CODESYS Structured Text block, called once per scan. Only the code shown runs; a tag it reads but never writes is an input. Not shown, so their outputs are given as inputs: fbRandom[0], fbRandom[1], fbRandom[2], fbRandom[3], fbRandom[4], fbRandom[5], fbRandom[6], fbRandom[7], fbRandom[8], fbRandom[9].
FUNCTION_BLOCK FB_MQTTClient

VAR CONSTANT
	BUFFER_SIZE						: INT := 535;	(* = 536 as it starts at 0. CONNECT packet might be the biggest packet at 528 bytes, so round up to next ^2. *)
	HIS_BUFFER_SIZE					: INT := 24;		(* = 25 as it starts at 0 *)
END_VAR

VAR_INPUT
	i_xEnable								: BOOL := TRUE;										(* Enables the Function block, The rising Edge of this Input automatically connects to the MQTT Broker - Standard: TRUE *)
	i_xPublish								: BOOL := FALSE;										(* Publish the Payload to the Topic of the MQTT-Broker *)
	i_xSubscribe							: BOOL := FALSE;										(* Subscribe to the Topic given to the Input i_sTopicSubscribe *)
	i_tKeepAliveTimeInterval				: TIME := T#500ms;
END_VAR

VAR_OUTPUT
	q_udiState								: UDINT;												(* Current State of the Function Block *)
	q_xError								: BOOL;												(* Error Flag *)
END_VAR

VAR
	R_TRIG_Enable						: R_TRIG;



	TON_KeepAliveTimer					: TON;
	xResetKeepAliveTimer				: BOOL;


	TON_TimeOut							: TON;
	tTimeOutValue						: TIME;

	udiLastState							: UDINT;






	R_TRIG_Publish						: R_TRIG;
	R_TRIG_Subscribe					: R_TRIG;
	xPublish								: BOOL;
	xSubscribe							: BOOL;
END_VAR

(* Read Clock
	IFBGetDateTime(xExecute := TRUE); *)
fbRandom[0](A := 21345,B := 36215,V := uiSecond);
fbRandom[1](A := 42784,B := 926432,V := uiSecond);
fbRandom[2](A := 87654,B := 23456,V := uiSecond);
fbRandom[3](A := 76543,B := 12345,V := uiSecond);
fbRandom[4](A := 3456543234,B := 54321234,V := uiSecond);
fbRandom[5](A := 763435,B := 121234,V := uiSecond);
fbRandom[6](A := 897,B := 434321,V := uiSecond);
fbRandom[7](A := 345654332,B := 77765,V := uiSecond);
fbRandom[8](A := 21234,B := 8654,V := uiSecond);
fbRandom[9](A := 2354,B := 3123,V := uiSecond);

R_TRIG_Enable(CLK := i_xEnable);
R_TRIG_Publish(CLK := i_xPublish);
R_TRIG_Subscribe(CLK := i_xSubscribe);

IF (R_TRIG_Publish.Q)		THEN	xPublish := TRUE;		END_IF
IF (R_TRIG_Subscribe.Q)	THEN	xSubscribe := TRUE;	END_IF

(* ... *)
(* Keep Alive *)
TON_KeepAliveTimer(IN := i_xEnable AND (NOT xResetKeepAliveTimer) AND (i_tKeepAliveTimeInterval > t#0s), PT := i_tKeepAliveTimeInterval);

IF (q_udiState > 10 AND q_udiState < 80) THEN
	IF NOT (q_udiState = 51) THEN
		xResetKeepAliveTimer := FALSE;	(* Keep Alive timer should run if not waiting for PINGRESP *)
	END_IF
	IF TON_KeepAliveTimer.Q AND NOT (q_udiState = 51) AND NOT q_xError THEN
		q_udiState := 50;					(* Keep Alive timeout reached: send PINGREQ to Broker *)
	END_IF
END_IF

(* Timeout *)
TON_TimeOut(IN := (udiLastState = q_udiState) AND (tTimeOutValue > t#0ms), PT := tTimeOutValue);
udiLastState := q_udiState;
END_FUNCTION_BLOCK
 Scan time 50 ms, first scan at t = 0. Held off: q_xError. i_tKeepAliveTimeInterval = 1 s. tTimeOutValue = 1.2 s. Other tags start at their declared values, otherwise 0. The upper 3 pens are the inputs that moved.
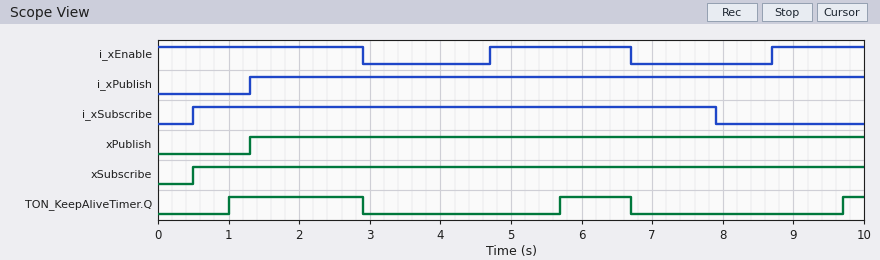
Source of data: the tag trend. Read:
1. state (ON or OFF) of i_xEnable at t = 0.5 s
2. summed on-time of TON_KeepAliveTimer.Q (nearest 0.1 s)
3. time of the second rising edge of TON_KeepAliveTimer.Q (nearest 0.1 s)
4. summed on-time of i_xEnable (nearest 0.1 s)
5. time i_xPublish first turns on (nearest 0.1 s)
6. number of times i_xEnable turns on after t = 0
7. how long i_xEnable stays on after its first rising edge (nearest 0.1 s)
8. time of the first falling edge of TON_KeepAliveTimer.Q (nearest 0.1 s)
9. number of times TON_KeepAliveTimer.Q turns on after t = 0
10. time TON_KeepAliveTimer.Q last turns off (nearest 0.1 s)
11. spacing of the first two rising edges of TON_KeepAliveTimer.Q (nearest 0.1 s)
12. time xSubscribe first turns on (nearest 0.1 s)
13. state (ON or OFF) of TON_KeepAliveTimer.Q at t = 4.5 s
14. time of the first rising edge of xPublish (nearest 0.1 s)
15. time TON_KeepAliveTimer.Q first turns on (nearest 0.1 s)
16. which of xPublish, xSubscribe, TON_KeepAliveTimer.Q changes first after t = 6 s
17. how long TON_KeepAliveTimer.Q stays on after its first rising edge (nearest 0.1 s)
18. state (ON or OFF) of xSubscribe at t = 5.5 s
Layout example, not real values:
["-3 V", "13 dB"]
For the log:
["ON", "3.2 s", "5.7 s", "6.2 s", "1.3 s", "2", "2.0 s", "2.9 s", "3", "6.7 s", "4.7 s", "0.5 s", "OFF", "1.3 s", "1.0 s", "TON_KeepAliveTimer.Q", "1.9 s", "ON"]
